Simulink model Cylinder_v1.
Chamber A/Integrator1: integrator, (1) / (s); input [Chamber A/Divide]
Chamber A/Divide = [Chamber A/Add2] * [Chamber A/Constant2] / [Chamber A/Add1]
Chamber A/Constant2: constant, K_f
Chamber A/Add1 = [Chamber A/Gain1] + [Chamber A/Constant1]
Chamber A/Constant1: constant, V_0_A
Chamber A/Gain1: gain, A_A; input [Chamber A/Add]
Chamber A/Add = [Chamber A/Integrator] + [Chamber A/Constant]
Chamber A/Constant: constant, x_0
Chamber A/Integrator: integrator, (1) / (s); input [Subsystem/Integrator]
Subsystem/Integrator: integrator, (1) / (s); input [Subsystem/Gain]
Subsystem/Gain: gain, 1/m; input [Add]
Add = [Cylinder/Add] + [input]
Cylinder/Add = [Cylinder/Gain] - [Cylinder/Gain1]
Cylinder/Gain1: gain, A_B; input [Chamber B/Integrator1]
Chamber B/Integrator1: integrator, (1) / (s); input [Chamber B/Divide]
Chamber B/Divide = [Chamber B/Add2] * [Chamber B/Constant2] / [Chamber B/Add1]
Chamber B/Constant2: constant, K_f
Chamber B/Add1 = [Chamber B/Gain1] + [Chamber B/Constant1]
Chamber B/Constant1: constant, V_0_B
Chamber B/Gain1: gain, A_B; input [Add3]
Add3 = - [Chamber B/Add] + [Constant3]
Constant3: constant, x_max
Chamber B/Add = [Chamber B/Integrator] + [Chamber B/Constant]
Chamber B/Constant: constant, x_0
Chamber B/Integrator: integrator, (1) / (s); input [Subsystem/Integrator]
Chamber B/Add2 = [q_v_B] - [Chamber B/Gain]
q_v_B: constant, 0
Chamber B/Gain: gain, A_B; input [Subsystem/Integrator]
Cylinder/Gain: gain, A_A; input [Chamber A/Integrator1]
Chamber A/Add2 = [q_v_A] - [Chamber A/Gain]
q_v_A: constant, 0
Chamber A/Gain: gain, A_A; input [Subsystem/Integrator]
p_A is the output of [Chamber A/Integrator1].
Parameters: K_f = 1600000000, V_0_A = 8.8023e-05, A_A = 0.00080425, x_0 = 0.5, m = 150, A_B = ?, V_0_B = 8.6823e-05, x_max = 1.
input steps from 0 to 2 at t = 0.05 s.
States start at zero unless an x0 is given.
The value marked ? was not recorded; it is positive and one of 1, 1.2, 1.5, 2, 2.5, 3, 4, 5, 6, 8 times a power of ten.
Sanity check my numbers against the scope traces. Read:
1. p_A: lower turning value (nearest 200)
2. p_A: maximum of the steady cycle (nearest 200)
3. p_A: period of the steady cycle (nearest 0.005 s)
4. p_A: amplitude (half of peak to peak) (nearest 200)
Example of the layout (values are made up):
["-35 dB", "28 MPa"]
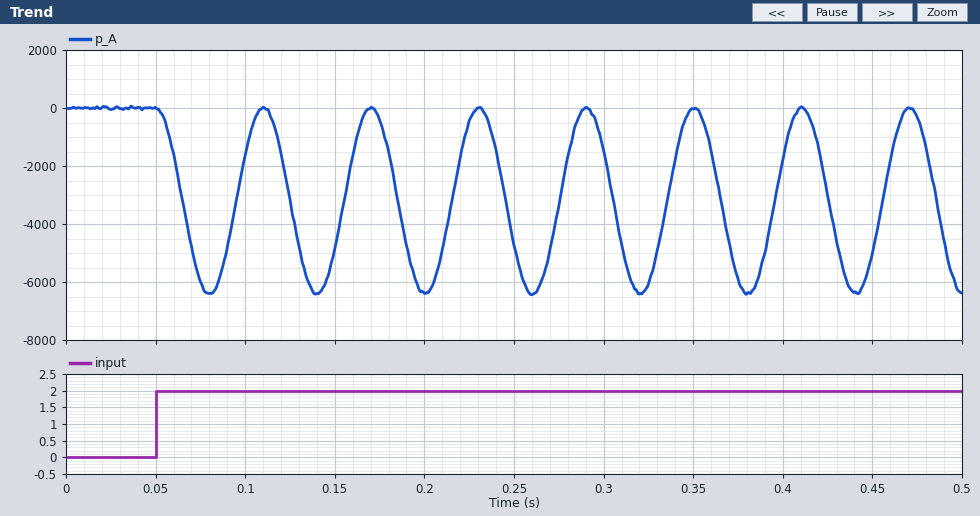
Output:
["-6400", "0", "0.060 s", "3200"]
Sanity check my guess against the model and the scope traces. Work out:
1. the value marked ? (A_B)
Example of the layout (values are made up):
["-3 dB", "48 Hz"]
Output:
["0.00025"]
